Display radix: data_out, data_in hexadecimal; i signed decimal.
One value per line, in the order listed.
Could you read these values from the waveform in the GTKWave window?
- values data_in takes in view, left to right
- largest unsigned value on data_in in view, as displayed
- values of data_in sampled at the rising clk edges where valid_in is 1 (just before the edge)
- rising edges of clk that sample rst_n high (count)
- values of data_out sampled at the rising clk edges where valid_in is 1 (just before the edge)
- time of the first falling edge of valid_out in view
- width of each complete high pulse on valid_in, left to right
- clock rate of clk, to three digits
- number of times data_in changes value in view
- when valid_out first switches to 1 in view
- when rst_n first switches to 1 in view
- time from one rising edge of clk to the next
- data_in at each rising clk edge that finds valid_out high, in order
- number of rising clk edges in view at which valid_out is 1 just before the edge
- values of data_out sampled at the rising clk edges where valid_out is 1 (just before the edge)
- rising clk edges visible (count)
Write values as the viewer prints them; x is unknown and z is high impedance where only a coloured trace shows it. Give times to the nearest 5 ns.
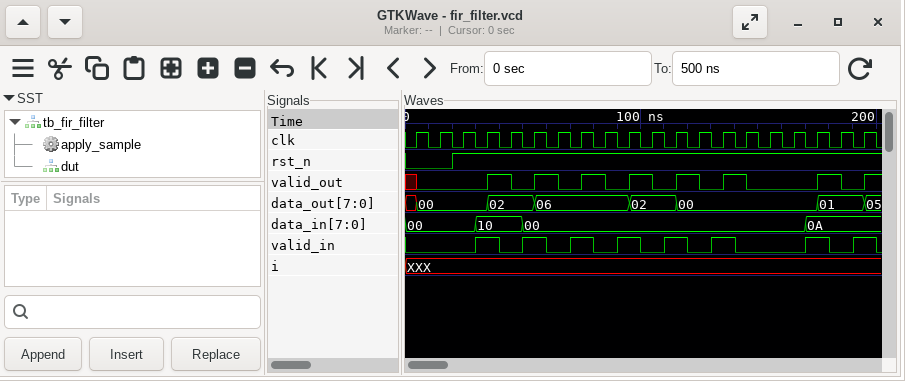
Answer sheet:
00, 10, 00, 0A
10
10, 00, 00, 00, 00, 00, 0A, 0A
18
00, 02, 06, 06, 02, 00, 00, 01
45 ns
10 ns, 10 ns, 10 ns, 10 ns, 10 ns, 10 ns, 10 ns, 10 ns
100 MHz
3
35 ns
20 ns
10 ns
10, 00, 00, 00, 00, 00, 0A
7
02, 06, 06, 02, 00, 00, 01
20
